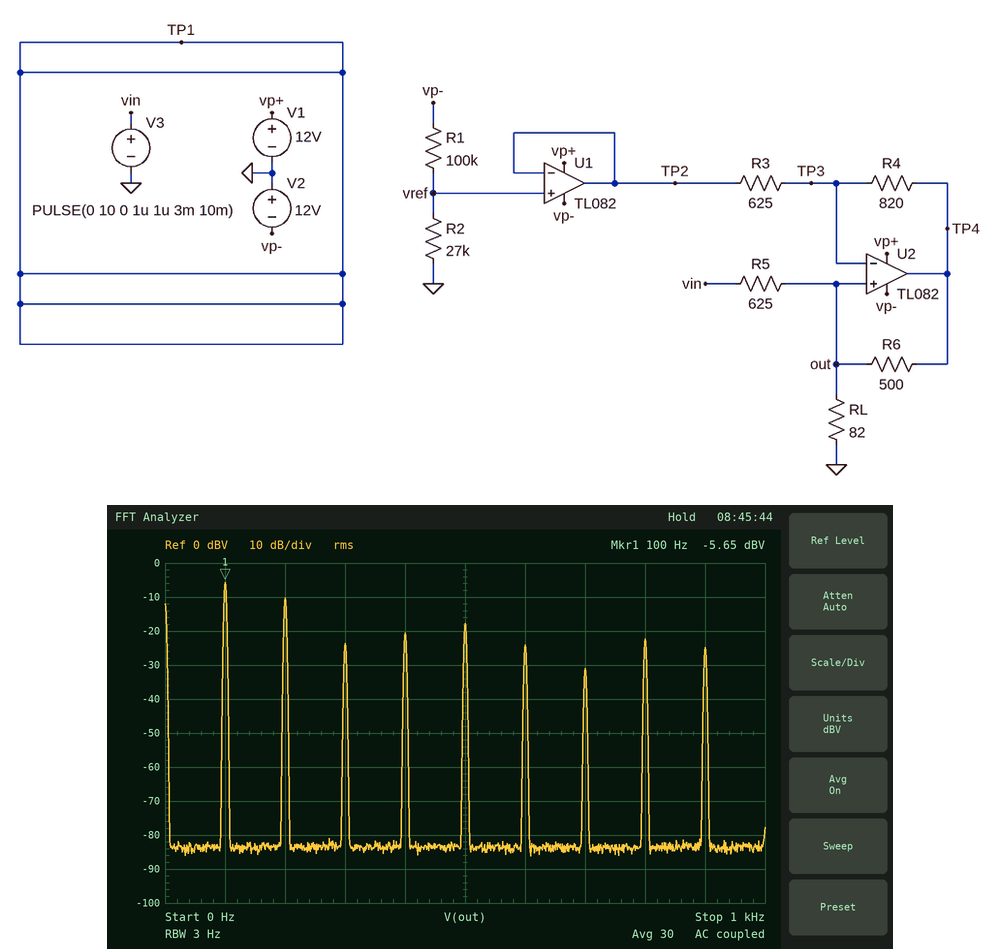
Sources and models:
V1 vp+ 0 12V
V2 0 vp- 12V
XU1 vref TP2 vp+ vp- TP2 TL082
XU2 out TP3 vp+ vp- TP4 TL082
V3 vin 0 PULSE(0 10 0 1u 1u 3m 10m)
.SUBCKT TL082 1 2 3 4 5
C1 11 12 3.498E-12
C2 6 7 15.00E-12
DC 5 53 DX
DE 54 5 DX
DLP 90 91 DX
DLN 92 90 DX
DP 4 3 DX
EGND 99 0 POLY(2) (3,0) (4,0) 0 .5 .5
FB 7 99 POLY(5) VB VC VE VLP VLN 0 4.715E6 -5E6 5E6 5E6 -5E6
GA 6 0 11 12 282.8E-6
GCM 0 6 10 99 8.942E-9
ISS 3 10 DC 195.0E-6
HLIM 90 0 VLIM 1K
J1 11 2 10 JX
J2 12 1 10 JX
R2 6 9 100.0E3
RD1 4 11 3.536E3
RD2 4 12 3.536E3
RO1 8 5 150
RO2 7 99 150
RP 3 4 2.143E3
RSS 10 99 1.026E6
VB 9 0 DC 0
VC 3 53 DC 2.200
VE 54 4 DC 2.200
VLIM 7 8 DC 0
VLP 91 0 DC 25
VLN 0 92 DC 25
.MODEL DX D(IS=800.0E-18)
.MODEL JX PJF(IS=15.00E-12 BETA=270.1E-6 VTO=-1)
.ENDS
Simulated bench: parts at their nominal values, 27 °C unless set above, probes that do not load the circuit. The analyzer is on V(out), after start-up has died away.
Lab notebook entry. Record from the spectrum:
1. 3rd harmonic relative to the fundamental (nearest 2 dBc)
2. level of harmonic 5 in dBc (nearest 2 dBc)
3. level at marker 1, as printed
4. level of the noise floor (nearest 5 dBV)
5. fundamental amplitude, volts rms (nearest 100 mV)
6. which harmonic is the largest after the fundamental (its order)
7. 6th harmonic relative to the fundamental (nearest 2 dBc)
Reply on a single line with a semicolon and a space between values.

-18 dBc; -12 dBc; -5.65 dBV; -85 dBV; 500 mV; 2; -18 dBc
